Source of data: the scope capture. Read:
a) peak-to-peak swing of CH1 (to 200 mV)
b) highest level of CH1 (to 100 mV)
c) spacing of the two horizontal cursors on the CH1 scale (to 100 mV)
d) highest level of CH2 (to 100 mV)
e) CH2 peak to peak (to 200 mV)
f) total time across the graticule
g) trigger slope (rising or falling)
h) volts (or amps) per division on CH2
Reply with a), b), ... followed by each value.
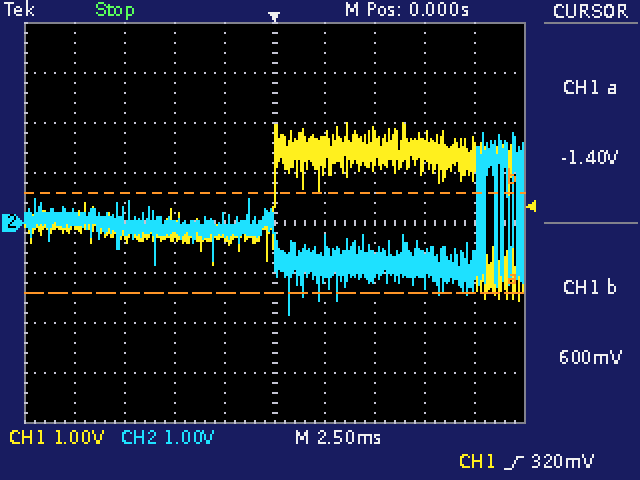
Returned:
a) 3.6 V
b) 2.0 V
c) 2.0 V
d) 1.8 V
e) 3.6 V
f) 25 ms
g) rising
h) 1 V
